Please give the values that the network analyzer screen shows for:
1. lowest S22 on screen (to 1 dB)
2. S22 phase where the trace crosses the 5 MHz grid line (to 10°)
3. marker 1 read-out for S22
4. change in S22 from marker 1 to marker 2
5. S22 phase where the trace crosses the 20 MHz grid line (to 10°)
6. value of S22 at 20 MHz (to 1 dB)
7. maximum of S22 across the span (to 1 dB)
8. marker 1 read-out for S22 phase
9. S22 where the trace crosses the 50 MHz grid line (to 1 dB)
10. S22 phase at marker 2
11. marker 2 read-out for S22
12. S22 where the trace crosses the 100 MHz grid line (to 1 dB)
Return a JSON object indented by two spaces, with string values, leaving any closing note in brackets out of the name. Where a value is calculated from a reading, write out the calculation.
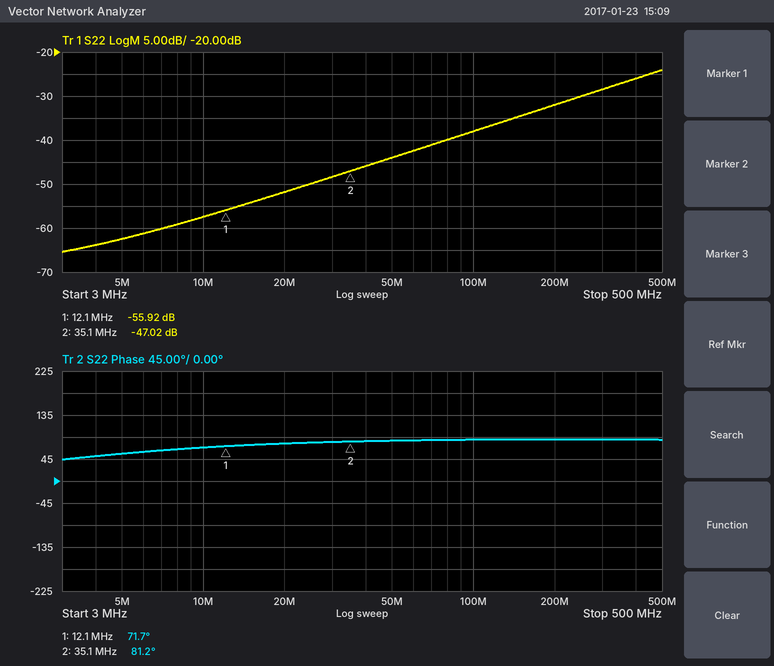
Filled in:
{
  "lowest S22 on screen": "-65 dB",
  "S22 phase where the trace crosses the 5 MHz grid line": "60°",
  "marker 1 read-out for S22": "-55.92 dB",
  "change in S22 from marker 1 to marker 2": "-47.02 − (-55.92) = 8.90 dB",
  "S22 phase where the trace crosses the 20 MHz grid line": "80°",
  "value of S22 at 20 MHz": "-52 dB",
  "maximum of S22 across the span": "-24 dB",
  "marker 1 read-out for S22 phase": "71.7°",
  "S22 where the trace crosses the 50 MHz grid line": "-44 dB",
  "S22 phase at marker 2": "81.2°",
  "marker 2 read-out for S22": "-47.02 dB",
  "S22 where the trace crosses the 100 MHz grid line": "-38 dB"
}
